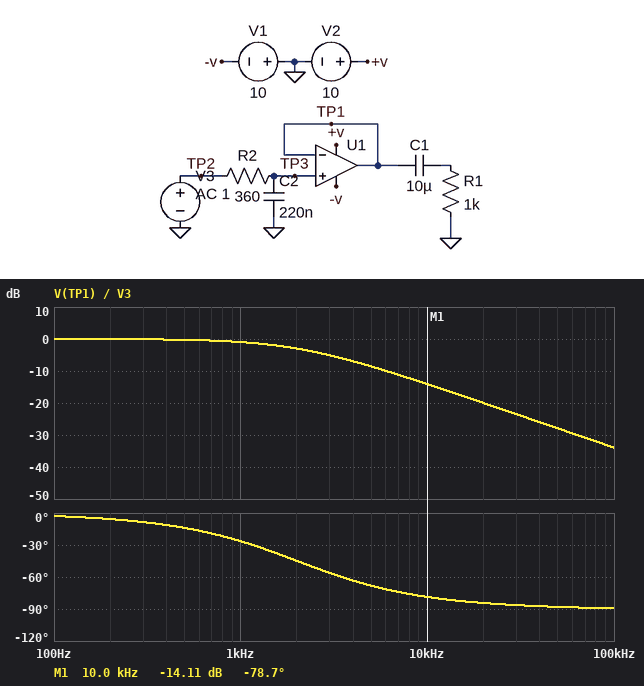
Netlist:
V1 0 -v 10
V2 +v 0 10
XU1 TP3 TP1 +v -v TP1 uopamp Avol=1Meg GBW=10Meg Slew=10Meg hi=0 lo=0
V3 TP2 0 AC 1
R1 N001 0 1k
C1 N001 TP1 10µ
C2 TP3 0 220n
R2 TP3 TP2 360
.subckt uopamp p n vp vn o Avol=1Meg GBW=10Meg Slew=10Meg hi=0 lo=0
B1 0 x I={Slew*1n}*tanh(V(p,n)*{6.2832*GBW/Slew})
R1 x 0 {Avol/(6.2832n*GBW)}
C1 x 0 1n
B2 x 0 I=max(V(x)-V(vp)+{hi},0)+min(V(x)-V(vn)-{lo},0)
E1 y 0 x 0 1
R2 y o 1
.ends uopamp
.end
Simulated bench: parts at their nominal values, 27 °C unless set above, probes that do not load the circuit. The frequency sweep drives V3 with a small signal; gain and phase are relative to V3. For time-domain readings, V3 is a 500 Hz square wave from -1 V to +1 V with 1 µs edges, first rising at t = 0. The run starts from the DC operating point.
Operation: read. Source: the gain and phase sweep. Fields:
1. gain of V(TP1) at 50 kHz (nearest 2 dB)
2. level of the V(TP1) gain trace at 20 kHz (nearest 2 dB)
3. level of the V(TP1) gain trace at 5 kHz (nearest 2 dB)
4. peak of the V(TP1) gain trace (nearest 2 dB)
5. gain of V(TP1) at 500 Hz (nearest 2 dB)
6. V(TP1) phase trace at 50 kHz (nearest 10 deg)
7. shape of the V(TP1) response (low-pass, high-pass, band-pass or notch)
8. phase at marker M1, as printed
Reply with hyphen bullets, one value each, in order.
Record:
- -28 dB
- -20 dB
- -8 dB
- 0 dB
- 0 dB
- -90 deg
- low-pass
- -78.7 deg
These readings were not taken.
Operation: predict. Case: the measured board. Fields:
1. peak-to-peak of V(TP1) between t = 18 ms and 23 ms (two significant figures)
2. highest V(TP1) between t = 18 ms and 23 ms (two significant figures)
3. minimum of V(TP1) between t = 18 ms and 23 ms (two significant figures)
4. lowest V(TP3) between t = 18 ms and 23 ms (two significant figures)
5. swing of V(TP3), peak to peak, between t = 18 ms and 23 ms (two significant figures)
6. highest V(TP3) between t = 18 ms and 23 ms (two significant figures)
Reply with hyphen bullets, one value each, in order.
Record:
- 2.0 V
- 1.0 V
- -1.0 V
- -1.0 V
- 2.0 V
- 1.0 V
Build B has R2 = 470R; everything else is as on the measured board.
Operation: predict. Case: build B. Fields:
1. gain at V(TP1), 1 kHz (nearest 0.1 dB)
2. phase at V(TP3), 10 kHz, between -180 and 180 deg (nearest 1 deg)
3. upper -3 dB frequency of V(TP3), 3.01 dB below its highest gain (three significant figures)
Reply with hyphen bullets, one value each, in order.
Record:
- -1.5 dB
- -81 deg
- 1.54 kHz
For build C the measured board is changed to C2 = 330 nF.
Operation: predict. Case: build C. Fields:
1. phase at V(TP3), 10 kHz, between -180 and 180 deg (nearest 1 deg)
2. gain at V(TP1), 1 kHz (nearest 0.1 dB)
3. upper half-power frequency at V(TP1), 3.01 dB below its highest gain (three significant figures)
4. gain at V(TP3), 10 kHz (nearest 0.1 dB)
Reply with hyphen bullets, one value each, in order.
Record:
- -82 deg
- -1.9 dB
- 1.34 kHz
- -17.5 dB
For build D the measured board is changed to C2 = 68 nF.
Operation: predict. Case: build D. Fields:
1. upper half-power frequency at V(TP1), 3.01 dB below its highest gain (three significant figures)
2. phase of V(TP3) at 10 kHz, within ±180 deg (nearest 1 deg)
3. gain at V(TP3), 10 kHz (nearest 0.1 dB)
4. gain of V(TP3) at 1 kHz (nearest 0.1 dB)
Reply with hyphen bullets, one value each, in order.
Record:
- 6.50 kHz
- -57 deg
- -5.3 dB
- -0.1 dB
